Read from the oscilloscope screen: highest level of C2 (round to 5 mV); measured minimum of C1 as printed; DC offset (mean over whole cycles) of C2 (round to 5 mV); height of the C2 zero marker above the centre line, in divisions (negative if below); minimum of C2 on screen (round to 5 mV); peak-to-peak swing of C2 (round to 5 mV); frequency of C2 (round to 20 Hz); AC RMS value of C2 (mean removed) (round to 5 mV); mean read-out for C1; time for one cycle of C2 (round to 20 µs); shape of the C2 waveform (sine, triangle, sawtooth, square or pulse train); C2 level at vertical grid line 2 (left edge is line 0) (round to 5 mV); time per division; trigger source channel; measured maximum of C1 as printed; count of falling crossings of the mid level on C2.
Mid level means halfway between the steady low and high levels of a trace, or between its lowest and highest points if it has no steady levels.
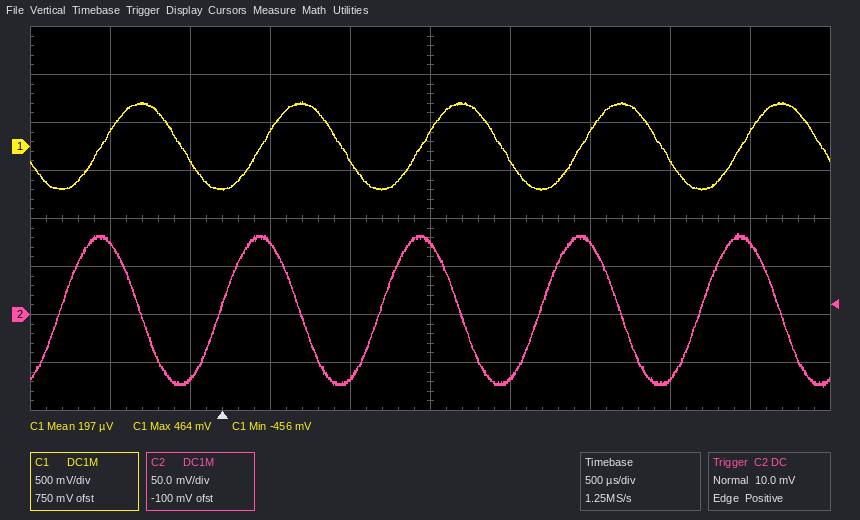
85 mV
-456 mV
5 mV
-2.0 div
-75 mV
160 mV
1.00 kHz
55 mV
197 µV
1.00 ms
sine
-65 mV
500 µs
C2
464 mV
5
